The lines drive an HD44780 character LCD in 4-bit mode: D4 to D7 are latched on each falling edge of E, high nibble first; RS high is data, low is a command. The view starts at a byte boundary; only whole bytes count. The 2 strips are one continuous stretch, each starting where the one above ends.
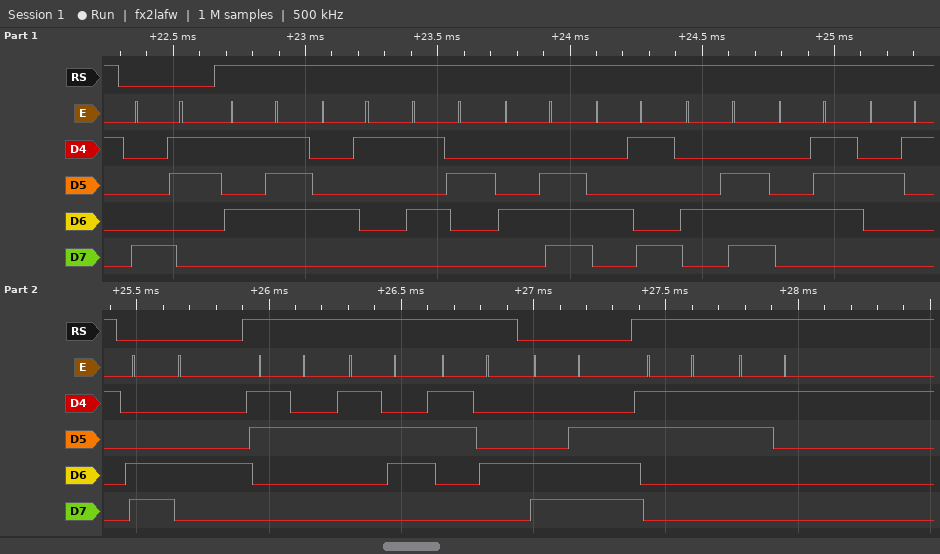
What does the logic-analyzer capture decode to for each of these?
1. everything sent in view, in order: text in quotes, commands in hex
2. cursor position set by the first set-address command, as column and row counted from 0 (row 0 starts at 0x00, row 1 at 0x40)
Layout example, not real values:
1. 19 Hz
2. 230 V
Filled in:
1. 0x83 "WARNING!" 0xC4 "264" 0xCE "31"
2. column 3, row 0
